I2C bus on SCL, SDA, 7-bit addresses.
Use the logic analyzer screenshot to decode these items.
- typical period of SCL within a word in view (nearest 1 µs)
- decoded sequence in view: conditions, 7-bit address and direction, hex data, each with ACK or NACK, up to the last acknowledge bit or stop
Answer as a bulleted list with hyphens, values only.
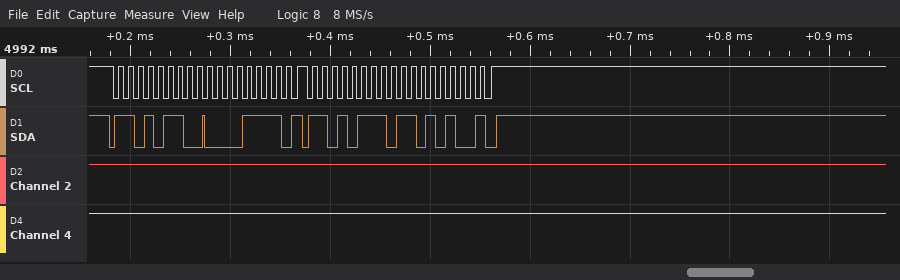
- 10 µs
- start, address 6B write ACK, 0F ACK, repeated start, address 6B read ACK, D4 NACK, stop
